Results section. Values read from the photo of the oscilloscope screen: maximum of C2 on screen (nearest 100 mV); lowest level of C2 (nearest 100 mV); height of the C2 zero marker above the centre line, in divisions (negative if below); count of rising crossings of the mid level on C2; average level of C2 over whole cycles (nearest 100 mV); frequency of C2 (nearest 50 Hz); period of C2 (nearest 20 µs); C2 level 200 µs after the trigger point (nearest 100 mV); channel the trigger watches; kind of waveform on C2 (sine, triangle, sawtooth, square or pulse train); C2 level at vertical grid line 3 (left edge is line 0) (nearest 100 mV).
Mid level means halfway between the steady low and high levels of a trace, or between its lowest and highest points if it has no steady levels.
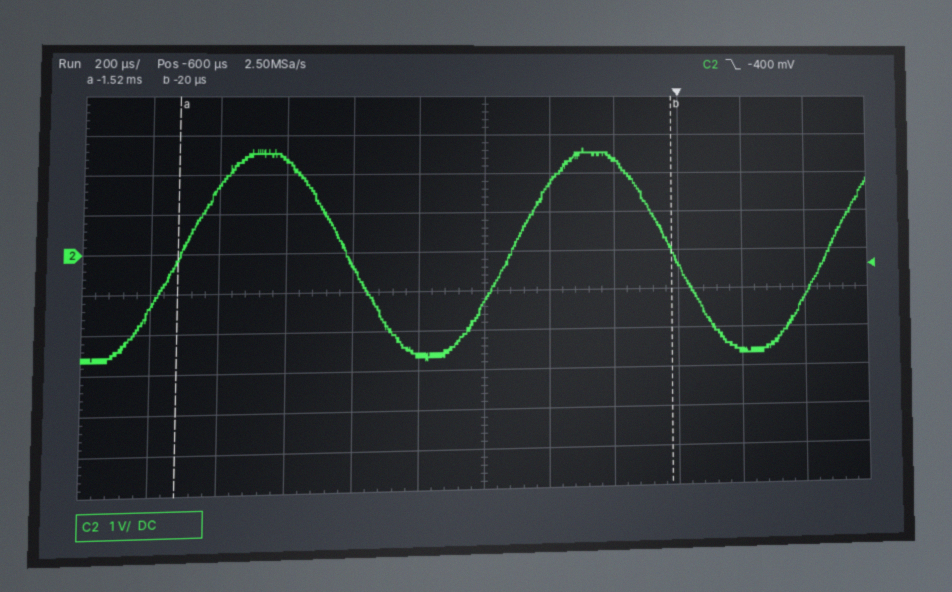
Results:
2.6 V
-2.7 V
+1.0 div
3
0.0 V
1.00 kHz
1.00 ms
-2.6 V
C2
sine
2.4 V
